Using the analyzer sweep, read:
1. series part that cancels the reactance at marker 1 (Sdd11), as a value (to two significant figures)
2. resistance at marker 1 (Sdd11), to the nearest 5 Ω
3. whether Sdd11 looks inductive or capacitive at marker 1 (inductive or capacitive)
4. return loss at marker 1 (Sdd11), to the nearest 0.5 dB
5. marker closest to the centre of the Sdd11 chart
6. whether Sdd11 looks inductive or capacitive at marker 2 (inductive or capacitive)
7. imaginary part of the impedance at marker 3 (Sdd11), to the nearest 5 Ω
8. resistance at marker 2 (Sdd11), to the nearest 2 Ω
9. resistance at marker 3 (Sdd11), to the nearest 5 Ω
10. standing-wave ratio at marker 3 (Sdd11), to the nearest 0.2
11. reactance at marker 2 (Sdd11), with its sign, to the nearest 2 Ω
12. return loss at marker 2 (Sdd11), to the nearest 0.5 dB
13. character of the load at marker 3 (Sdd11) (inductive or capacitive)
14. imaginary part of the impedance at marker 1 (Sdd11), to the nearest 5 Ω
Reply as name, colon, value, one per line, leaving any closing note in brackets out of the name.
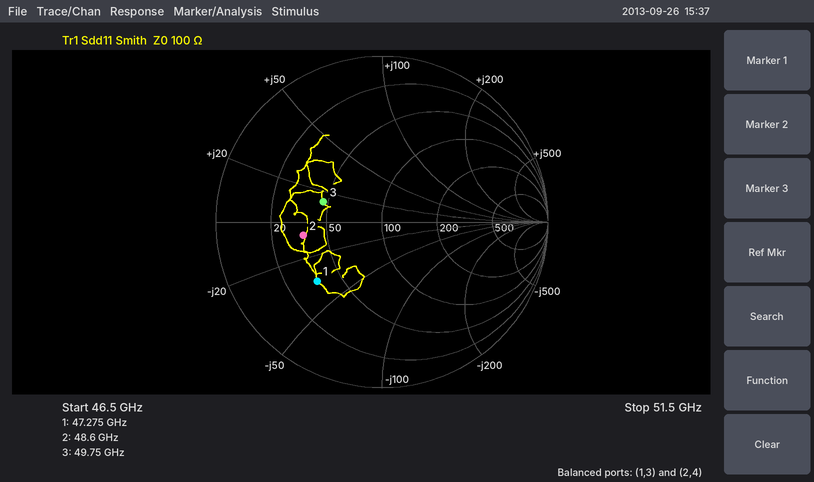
series part that cancels the reactance at marker 1 (Sdd11), as a value: 120 pH
resistance at marker 1 (Sdd11), to the nearest 5 Ω: 35 Ω
whether Sdd11 looks inductive or capacitive at marker 1: capacitive
return loss at marker 1 (Sdd11), to the nearest 0.5 dB: 5.5 dB
marker closest to the centre of the Sdd11 chart: marker 3
whether Sdd11 looks inductive or capacitive at marker 2: capacitive
imaginary part of the impedance at marker 3 (Sdd11), to the nearest 5 Ω: +15 Ω
resistance at marker 2 (Sdd11), to the nearest 2 Ω: 36 Ω
resistance at marker 3 (Sdd11), to the nearest 5 Ω: 45 Ω
standing-wave ratio at marker 3 (Sdd11), to the nearest 0.2: 2.2
reactance at marker 2 (Sdd11), with its sign, to the nearest 2 Ω: -8 Ω
return loss at marker 2 (Sdd11), to the nearest 0.5 dB: 6.5 dB
character of the load at marker 3 (Sdd11): inductive
imaginary part of the impedance at marker 1 (Sdd11), to the nearest 5 Ω: -35 Ω
